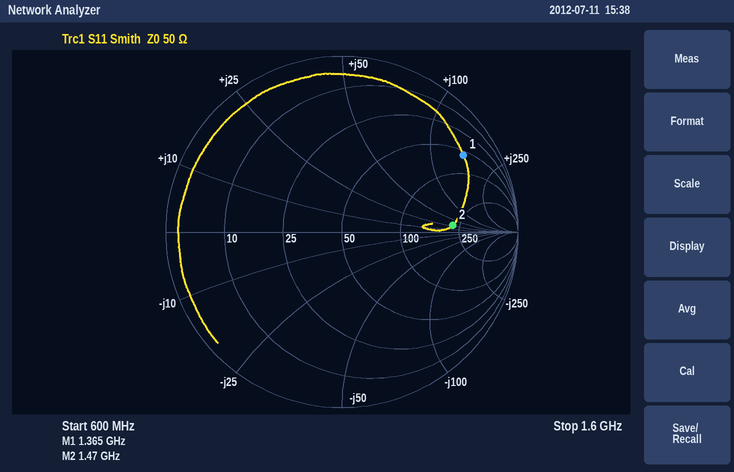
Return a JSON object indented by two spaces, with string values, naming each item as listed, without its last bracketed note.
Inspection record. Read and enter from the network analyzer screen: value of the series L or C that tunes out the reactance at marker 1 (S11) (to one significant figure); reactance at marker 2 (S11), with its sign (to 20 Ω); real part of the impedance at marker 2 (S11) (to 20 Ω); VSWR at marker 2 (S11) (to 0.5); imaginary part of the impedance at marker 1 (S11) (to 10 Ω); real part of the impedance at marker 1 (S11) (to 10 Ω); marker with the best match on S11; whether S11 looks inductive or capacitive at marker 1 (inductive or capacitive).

{
  "value of the series L or C that tunes out the reactance at marker 1 (S11)": "800 fF",
  "reactance at marker 2 (S11), with its sign": "+20 Ω",
  "real part of the impedance at marker 2 (S11)": "220 Ω",
  "VSWR at marker 2 (S11)": "4.5",
  "imaginary part of the impedance at marker 1 (S11)": "+150 Ω",
  "real part of the impedance at marker 1 (S11)": "60 Ω",
  "marker with the best match on S11": "marker 2",
  "whether S11 looks inductive or capacitive at marker 1": "inductive"
}
